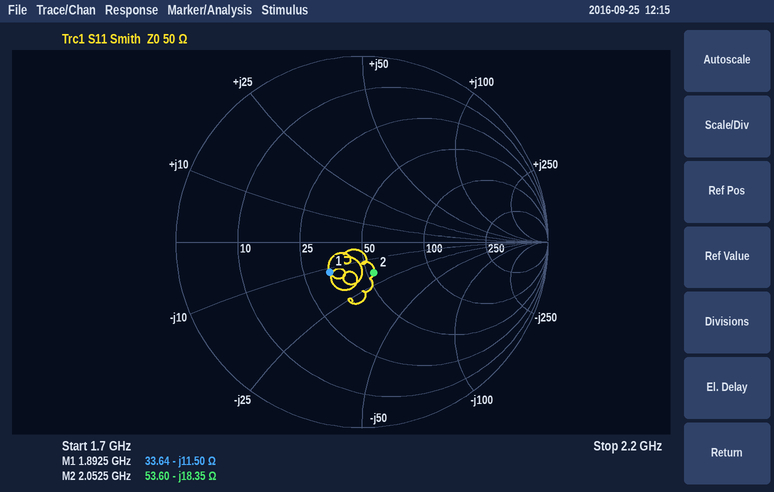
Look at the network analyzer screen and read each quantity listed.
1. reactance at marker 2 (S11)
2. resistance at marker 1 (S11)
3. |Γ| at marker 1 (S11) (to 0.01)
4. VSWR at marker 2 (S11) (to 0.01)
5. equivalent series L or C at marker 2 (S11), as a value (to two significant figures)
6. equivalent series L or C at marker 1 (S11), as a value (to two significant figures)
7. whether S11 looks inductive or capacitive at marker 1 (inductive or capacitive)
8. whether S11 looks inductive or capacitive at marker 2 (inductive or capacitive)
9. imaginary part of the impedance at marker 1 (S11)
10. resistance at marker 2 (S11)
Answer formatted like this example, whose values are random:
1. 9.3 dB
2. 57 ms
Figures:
1. -18.35 Ω
2. 33.64 Ω
3. 0.24
4. 1.43
5. 4.2 pF
6. 7.3 pF
7. capacitive
8. capacitive
9. -11.50 Ω
10. 53.60 Ω
